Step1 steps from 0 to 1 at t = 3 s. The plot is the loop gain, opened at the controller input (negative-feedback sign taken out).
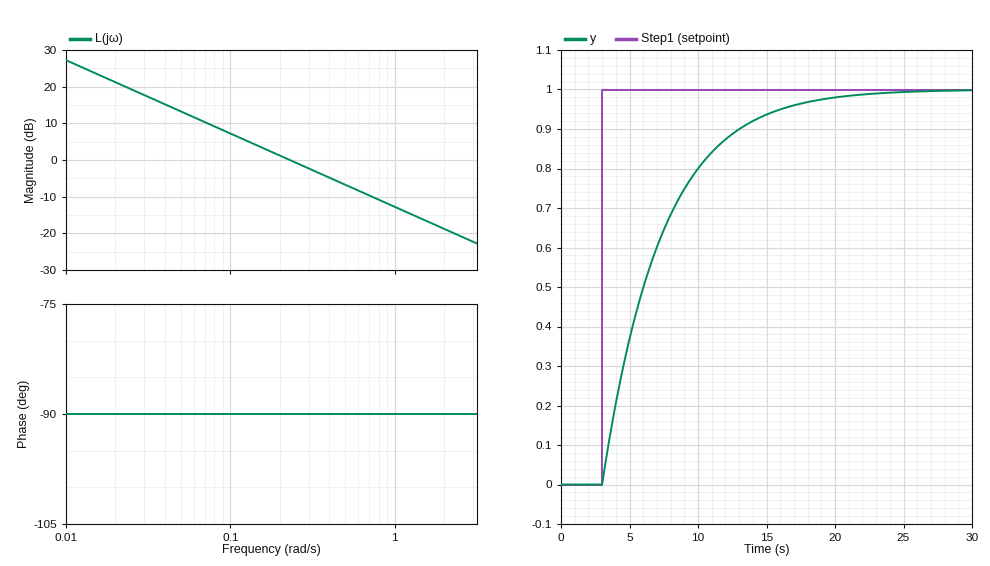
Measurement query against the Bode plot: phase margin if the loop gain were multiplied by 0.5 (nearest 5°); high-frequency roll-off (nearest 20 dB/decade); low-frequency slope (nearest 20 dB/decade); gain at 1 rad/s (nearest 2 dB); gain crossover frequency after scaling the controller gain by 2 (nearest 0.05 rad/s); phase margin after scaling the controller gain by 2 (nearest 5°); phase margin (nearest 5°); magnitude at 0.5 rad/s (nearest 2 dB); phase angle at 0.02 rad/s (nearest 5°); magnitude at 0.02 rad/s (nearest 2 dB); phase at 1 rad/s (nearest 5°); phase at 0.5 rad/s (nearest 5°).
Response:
90°
-20 dB/decade
-20 dB/decade
-12 dB
0.45 rad/s
90°
90°
-6 dB
-90°
22 dB
-90°
-90°
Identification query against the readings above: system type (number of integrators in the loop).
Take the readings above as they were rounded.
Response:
1
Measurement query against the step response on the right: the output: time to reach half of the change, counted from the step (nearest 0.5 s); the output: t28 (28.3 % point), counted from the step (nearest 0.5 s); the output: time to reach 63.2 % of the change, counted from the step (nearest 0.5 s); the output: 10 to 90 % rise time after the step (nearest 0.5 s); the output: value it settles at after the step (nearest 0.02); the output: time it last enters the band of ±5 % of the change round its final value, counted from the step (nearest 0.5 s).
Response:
3.0 s
1.5 s
4.5 s
9.5 s
1.00
13.0 s
